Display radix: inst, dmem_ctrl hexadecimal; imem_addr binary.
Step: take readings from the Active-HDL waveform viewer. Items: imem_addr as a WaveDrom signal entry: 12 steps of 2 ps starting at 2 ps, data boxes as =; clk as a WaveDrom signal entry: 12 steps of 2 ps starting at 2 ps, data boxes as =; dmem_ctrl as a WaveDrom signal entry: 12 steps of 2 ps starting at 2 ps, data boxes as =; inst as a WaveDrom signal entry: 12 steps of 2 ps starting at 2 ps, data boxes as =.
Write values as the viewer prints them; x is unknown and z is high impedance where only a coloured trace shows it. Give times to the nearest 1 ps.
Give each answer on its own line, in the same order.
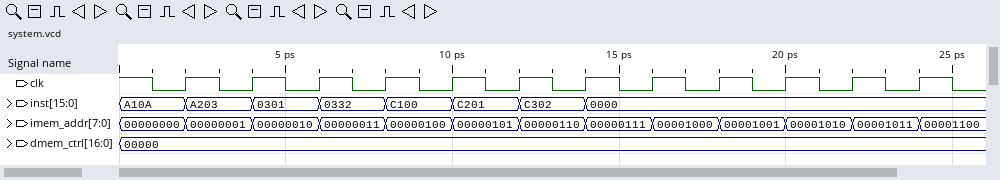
{name: 'imem_addr', wave: '============', data: '00000001 00000010 00000011 00000100 00000101 00000110 00000111 00001000 00001001 00001010 00001011 00001100'}
{name: 'clk', wave: 'p...........'}
{name: 'dmem_ctrl', wave: '=...........', data: '00000'}
{name: 'inst', wave: '=======.....', data: 'A203 0301 0332 C100 C201 C302 0000'}
